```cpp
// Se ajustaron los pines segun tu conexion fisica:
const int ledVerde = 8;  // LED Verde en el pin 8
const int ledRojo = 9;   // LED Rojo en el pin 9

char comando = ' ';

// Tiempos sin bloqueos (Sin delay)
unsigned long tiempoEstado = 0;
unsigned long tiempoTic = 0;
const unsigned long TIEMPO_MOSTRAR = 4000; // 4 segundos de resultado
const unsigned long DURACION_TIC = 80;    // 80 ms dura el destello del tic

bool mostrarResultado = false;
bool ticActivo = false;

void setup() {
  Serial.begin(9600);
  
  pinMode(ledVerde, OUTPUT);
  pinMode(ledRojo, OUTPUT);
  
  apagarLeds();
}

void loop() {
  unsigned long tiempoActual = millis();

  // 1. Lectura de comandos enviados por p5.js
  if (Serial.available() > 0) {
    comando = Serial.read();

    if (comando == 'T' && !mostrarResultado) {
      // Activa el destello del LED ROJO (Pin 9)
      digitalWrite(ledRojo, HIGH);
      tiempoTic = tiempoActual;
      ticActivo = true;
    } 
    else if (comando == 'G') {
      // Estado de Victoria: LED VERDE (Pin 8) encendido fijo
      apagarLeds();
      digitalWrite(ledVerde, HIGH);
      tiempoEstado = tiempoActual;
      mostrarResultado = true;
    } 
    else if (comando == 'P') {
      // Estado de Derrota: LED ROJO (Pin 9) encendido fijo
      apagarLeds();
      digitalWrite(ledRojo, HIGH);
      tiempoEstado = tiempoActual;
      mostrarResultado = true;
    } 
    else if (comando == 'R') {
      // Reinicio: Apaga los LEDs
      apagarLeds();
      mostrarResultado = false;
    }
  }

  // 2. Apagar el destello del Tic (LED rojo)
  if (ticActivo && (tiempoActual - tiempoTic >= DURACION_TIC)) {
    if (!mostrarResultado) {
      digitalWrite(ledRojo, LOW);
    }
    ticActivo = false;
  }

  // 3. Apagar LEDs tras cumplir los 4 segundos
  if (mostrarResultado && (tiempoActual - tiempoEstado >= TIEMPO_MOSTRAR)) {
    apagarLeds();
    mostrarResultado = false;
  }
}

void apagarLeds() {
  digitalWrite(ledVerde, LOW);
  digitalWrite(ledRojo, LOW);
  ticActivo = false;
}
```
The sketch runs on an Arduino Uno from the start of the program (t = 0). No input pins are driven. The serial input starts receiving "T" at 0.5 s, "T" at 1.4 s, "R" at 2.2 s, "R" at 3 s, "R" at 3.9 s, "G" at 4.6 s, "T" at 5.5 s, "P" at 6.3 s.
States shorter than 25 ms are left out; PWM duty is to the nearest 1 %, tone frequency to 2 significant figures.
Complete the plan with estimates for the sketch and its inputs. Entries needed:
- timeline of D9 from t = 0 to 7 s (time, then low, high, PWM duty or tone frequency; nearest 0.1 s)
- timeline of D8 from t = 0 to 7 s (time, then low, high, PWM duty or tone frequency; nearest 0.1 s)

0 s low; 0.5 s high; 0.6 s low; 1.4 s high; 1.5 s low; 6.3 s high
0 s low; 4.6 s high; 6.3 s low
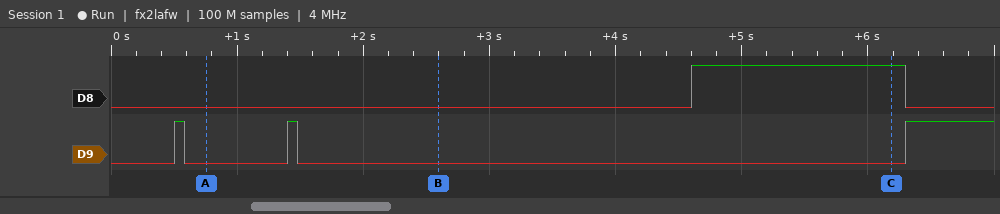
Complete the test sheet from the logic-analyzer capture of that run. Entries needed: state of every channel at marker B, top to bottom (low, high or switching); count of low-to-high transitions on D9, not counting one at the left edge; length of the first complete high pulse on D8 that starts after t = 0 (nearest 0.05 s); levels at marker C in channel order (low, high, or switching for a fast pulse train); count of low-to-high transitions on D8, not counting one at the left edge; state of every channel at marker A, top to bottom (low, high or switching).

D8 low, D9 low
3
1.70 s
D8 high, D9 low
1
D8 low, D9 low
